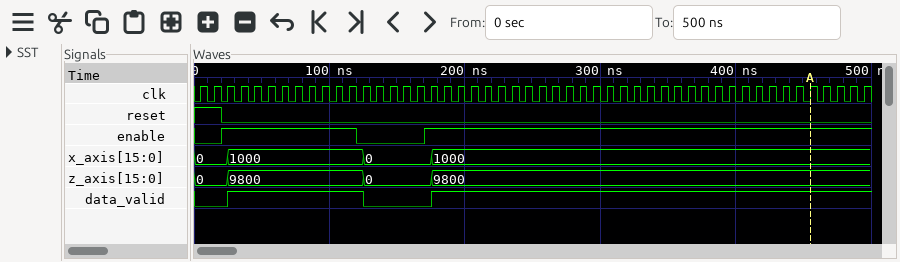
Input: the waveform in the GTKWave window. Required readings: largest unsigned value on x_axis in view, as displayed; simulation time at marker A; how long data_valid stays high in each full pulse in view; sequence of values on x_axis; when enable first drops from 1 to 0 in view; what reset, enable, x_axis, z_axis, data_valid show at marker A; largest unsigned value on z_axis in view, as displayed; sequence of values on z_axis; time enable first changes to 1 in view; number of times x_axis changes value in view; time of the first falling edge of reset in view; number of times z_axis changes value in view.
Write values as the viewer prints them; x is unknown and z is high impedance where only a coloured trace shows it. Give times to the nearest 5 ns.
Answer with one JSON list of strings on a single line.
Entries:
["1000", "455 ns", "100 ns", "0, 1000, 0, 1000", "120 ns", "reset=0, enable=1, x_axis=1000, z_axis=9800, data_valid=1", "9800", "0, 9800, 0, 9800", "20 ns", "3", "20 ns", "3"]
